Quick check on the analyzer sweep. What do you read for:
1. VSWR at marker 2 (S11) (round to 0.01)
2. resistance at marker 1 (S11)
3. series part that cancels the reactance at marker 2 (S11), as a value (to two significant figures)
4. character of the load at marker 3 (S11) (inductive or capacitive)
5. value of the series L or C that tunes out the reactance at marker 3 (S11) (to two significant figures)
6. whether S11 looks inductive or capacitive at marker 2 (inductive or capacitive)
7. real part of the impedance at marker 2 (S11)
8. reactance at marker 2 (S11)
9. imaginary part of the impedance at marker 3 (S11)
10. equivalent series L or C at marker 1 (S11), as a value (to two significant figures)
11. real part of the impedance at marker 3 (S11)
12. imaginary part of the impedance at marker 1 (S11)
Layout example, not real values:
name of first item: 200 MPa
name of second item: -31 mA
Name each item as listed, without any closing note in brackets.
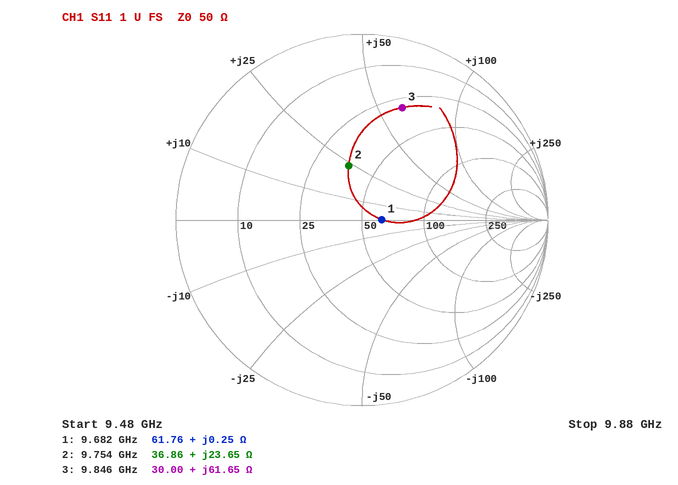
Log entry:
VSWR at marker 2 (S11): 1.86
resistance at marker 1: 61.76 Ω
series part that cancels the reactance at marker 2 (S11), as a value: 690 fF
character of the load at marker 3 (S11): inductive
value of the series L or C that tunes out the reactance at marker 3 (S11): 260 fF
whether S11 looks inductive or capacitive at marker 2: inductive
real part of the impedance at marker 2: 36.86 Ω
reactance at marker 2: +23.65 Ω
imaginary part of the impedance at marker 3: +61.65 Ω
equivalent series L or C at marker 1 (S11), as a value: 4.1 pH
real part of the impedance at marker 3: 30.00 Ω
imaginary part of the impedance at marker 1: +0.25 Ω
